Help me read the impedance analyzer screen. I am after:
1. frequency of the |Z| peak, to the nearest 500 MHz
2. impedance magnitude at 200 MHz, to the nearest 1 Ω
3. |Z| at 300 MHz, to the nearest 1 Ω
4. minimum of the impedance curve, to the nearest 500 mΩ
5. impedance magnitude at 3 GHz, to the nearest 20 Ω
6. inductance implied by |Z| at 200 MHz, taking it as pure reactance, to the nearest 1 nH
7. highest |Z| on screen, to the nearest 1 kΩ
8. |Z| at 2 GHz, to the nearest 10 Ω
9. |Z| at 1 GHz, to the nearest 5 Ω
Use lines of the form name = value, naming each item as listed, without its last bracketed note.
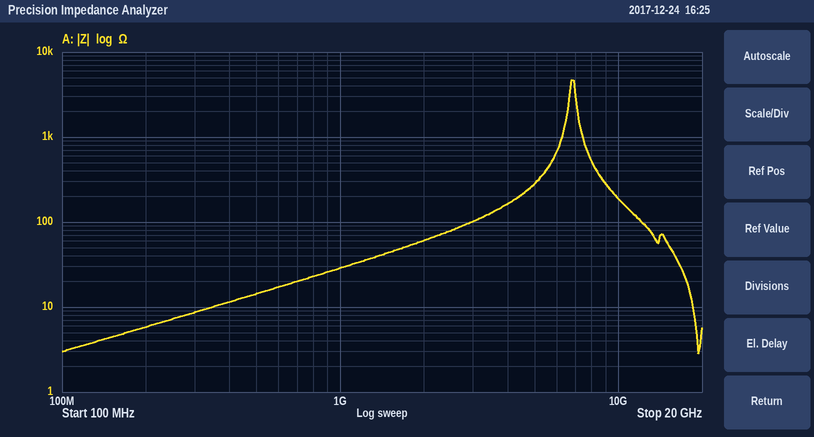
frequency of the |Z| peak, to the nearest 500 MHz = 7.0 GHz
impedance magnitude at 200 MHz, to the nearest 1 Ω = 6 Ω
|Z| at 300 MHz, to the nearest 1 Ω = 9 Ω
minimum of the impedance curve, to the nearest 500 mΩ = 3.0 Ω
impedance magnitude at 3 GHz, to the nearest 20 Ω = 100 Ω
inductance implied by |Z| at 200 MHz, taking it as pure reactance, to the nearest 1 nH = 5 nH
highest |Z| on screen, to the nearest 1 kΩ = 5 kΩ
|Z| at 2 GHz, to the nearest 10 Ω = 60 Ω
|Z| at 1 GHz, to the nearest 5 Ω = 30 Ω
